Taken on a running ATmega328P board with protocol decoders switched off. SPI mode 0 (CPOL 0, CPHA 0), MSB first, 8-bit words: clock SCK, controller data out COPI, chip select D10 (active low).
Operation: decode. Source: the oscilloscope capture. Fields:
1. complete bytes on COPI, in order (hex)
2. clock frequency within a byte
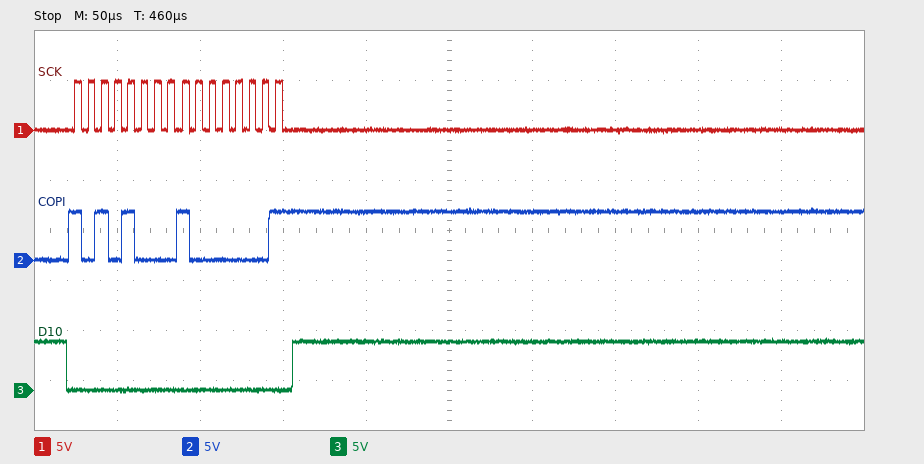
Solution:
A8 81
125 kHz
